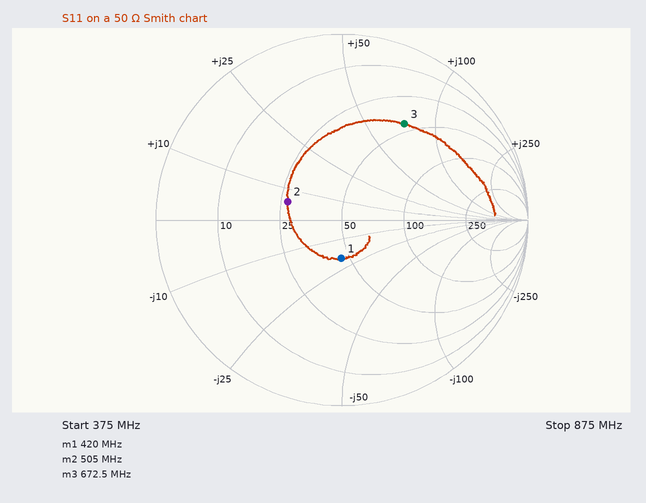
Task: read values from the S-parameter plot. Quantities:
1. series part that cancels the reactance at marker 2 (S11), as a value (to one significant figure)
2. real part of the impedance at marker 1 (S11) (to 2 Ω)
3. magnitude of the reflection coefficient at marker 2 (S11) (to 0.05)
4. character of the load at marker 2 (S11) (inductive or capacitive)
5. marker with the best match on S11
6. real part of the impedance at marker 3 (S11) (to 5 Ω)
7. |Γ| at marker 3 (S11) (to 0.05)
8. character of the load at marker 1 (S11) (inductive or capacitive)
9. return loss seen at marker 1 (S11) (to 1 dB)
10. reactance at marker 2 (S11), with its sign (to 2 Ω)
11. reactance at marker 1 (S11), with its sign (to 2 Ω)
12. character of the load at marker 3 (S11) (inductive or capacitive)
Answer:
50 pF
46 Ω
0.30
inductive
marker 1
45 Ω
0.60
capacitive
14 dB
+6 Ω
-20 Ω
inductive
